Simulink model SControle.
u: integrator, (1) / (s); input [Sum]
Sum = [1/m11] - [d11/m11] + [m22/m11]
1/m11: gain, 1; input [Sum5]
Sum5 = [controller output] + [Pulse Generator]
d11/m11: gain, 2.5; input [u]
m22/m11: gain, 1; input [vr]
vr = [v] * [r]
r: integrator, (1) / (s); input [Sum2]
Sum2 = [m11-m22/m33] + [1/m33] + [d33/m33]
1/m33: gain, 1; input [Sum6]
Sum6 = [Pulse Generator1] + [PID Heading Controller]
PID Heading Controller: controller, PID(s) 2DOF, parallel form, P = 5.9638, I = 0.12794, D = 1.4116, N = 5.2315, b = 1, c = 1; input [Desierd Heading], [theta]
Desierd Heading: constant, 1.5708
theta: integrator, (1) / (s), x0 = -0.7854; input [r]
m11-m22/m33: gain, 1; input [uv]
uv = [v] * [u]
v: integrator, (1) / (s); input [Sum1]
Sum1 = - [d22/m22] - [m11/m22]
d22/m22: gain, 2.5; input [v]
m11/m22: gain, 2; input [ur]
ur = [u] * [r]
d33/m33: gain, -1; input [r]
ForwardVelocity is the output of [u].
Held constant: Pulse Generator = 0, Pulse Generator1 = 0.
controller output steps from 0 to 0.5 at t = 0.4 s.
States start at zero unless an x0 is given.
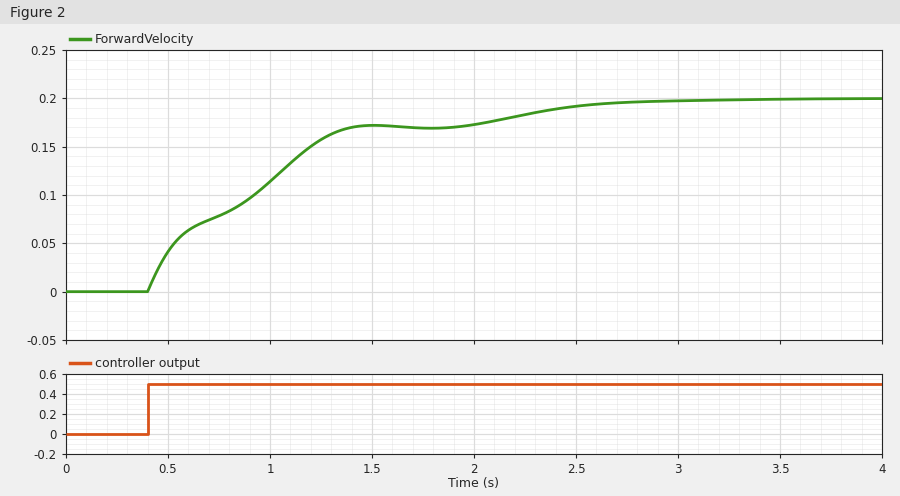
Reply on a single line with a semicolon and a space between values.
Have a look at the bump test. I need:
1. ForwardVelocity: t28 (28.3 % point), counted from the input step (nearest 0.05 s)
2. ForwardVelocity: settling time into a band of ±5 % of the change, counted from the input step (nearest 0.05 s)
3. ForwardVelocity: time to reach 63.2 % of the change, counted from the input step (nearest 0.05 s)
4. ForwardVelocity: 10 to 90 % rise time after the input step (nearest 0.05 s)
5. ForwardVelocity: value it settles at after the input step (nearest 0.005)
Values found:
0.15 s; 2.05 s; 0.65 s; 1.75 s; 0.200
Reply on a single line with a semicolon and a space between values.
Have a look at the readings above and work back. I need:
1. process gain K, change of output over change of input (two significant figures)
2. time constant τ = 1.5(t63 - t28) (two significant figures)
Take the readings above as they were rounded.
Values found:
0.40; 0.75 s
